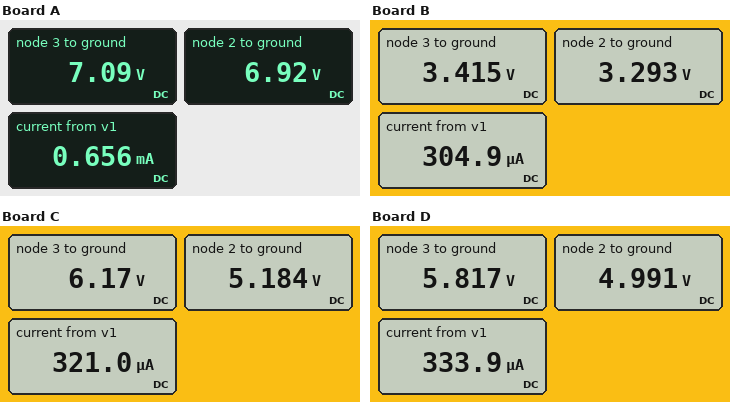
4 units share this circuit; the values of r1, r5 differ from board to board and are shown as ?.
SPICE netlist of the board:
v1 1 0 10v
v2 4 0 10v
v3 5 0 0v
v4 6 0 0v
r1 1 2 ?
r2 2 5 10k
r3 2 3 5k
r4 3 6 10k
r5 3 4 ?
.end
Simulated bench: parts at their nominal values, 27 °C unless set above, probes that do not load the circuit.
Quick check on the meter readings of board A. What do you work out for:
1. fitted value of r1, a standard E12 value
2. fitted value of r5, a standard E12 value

4.7 kΩ
3.9 kΩ
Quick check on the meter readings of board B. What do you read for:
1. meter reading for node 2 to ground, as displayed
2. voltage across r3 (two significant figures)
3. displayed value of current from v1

3.293 V
120 mV
304.9 µA
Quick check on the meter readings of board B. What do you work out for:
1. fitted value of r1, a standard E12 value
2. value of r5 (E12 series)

22 kΩ
18 kΩ
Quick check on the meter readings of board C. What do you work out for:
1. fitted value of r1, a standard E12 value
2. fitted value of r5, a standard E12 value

15 kΩ
4.7 kΩ
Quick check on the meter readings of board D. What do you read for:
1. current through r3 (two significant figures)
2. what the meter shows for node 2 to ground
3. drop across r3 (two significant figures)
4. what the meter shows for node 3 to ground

170 µA
4.991 V
830 mV
5.817 V
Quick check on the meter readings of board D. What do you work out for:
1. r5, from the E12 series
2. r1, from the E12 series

5.6 kΩ
15 kΩ
